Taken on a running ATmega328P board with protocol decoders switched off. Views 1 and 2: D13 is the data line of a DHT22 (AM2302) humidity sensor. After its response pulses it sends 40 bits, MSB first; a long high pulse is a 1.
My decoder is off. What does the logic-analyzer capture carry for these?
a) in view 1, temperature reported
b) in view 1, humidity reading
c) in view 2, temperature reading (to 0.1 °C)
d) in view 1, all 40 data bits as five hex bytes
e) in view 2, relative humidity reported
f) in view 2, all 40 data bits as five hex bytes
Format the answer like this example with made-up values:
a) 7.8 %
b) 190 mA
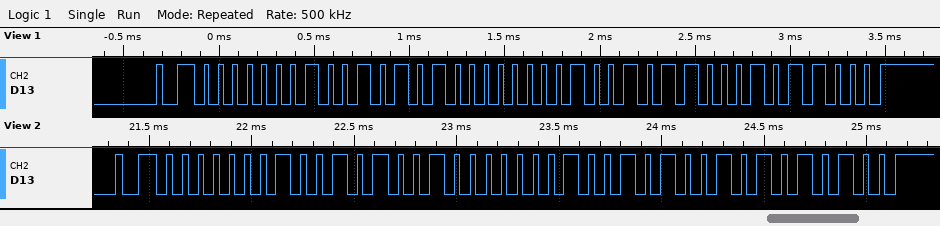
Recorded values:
a) 30.0 °C
b) 29.8 %
c) 29.7 °C
d) 01 2A 01 2C 58
e) 29.7 %
f) 01 29 01 29 54
